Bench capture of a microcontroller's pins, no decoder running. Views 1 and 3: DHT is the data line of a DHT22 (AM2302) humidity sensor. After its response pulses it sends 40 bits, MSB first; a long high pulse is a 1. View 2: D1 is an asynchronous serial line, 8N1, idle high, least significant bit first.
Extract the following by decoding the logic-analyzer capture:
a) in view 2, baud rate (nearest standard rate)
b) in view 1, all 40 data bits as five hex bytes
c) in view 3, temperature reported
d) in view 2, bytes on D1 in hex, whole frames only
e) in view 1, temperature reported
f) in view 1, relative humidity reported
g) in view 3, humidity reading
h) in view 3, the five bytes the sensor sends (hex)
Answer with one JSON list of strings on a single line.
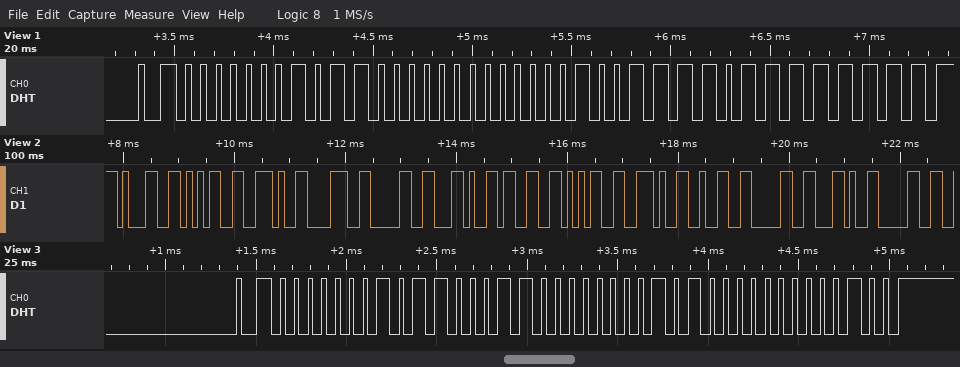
["9600 baud", "01 60 00 9E FF", "16.0 °C", "31 35 2E 38 30 2C 33 35 2E 32 30 2C 30", "15.8 °C", "35.2 %", "35.5 %", "01 63 00 A0 04"]
